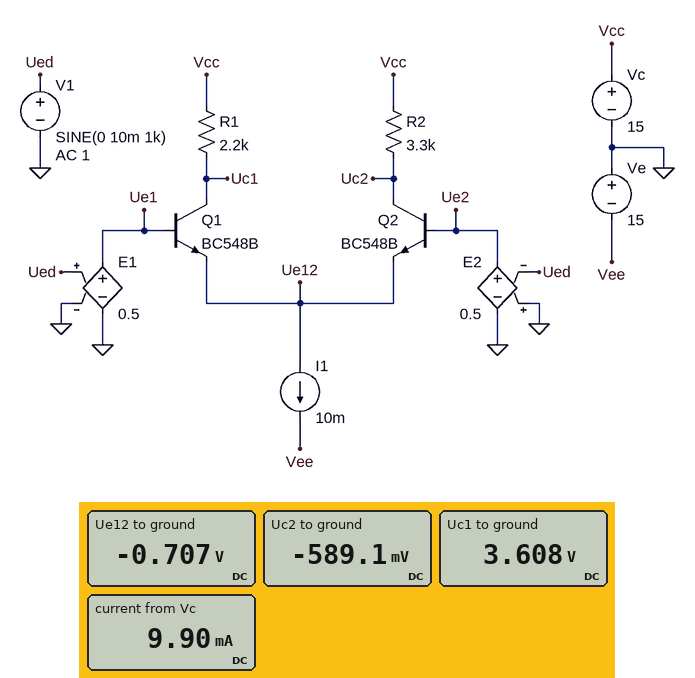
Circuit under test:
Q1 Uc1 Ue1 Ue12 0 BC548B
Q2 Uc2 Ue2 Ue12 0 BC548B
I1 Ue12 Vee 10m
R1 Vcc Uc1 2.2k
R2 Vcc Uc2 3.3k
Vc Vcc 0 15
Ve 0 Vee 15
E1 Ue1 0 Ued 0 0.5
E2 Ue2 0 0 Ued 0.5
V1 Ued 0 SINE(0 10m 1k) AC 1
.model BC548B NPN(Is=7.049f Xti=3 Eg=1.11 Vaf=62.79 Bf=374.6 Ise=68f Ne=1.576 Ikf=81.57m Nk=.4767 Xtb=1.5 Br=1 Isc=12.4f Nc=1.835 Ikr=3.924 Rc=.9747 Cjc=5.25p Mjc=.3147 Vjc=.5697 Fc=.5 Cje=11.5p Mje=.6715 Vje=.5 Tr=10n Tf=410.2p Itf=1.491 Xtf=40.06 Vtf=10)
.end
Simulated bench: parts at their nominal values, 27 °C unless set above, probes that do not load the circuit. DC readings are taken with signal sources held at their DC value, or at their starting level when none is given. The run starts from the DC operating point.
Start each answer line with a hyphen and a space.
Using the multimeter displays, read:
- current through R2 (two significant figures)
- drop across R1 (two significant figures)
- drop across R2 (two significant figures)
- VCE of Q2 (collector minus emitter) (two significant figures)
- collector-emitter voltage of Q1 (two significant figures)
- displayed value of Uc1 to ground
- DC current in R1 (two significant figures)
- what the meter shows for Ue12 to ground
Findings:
- 4.7 mA
- 11 V
- 16 V
- 120 mV
- 4.3 V
- 3.608 V
- 5.2 mA
- -0.707 V
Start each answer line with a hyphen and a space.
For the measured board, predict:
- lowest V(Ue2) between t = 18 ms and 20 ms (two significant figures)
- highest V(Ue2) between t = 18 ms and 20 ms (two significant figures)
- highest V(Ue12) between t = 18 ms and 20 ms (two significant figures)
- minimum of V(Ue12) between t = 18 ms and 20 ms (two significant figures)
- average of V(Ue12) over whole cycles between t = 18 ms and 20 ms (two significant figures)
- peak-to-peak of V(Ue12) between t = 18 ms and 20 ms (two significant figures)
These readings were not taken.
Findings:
- -5.0 mV
- 5.0 mV
- -710 mV
- -710 mV
- -710 mV
- 1.7 mV
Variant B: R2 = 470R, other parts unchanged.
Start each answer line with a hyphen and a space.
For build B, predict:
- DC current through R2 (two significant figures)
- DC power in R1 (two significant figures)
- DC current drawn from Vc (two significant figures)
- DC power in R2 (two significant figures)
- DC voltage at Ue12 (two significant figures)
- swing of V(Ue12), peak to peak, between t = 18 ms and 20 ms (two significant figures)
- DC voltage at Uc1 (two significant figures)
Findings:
- 5.3 mA
- 49 mW
- 10 mA
- 13 mW
- -700 mV
- 1.1 mV
- 4.6 V
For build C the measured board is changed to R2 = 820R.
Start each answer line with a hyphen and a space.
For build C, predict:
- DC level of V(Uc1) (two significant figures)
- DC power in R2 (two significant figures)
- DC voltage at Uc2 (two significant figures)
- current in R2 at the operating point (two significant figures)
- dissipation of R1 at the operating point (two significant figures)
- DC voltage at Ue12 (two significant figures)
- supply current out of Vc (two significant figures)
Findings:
- 4.5 V
- 22 mW
- 11 V
- 5.2 mA
- 50 mW
- -700 mV
- 10 mA
